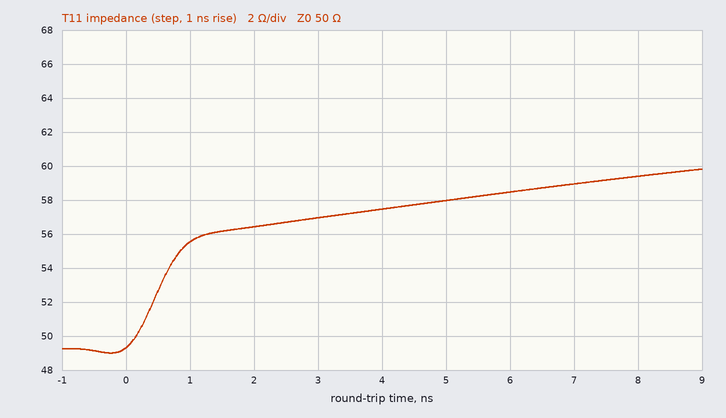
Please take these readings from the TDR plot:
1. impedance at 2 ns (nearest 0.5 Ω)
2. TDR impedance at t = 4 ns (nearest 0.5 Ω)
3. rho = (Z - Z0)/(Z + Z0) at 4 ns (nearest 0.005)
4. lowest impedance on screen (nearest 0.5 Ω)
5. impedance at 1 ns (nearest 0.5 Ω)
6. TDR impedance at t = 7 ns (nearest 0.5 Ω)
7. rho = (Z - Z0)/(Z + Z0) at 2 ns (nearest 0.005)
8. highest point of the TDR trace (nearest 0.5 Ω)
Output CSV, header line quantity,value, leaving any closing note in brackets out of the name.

quantity,value
impedance at 2 ns,56.5 Ω
TDR impedance at t = 4 ns,57.5 Ω
rho = (Z - Z0)/(Z + Z0) at 4 ns,+0.070
lowest impedance on screen,49.0 Ω
impedance at 1 ns,55.5 Ω
TDR impedance at t = 7 ns,59.0 Ω
rho = (Z - Z0)/(Z + Z0) at 2 ns,+0.060
highest point of the TDR trace,60.0 Ω
